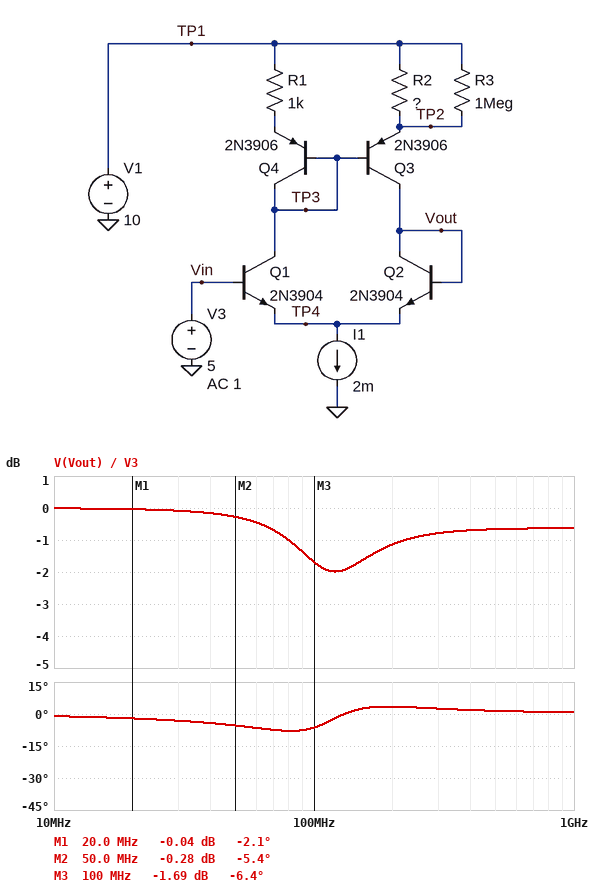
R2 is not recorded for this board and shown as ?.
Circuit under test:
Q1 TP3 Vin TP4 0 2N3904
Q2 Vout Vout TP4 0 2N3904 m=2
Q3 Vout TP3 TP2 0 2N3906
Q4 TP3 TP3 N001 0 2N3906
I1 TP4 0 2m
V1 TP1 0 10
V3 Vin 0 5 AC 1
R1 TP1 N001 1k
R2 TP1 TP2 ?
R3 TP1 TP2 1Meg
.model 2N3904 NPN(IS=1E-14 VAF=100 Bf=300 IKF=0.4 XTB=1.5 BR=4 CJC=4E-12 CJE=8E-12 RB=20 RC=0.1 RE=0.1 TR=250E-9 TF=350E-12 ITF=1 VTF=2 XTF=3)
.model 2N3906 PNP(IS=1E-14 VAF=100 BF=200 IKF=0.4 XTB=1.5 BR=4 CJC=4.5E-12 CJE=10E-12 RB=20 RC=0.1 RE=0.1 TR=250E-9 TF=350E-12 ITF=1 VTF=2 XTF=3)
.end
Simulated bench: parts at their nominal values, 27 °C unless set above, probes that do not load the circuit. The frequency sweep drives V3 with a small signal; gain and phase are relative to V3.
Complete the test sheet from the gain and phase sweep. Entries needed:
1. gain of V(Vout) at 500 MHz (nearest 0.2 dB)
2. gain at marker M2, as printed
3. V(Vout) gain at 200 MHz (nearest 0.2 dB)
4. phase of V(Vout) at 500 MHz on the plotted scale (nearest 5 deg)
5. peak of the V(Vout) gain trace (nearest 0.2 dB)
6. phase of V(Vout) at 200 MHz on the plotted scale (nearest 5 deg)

-0.6 dB
-0.28 dB
-1.2 dB
0 deg
0 dB
5 deg
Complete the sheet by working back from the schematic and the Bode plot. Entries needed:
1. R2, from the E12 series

470 Ω
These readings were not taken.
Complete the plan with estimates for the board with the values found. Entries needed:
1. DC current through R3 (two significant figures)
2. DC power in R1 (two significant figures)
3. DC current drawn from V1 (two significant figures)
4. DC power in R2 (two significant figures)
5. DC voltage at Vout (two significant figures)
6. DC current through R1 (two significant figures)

630 nA
420 µW
2.0 mA
850 µW
5.0 V
650 µA
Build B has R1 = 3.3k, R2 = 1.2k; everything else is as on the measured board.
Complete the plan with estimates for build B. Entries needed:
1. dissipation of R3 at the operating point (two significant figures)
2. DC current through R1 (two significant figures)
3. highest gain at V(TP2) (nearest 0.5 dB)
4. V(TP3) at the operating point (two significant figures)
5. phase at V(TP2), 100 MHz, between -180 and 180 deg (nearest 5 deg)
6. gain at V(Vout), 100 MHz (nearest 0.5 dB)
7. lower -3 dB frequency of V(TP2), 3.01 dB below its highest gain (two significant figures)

3.1 µW
540 µA
1.0 dB
7.6 V
20 deg
-1.0 dB
48 MHz
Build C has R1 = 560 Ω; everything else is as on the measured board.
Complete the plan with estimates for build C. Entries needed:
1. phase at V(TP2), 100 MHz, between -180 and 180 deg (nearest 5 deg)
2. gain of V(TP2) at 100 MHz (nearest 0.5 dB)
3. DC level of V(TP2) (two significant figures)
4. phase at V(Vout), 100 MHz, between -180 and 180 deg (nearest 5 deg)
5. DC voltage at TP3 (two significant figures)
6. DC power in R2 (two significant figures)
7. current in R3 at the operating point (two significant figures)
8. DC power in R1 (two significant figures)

80 deg
-4.5 dB
9.5 V
-5 deg
8.8 V
550 µW
510 nA
470 µW
